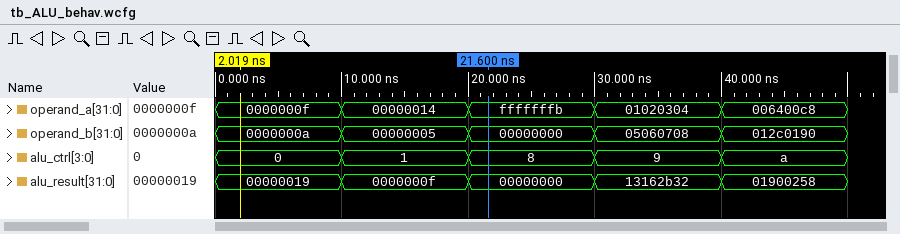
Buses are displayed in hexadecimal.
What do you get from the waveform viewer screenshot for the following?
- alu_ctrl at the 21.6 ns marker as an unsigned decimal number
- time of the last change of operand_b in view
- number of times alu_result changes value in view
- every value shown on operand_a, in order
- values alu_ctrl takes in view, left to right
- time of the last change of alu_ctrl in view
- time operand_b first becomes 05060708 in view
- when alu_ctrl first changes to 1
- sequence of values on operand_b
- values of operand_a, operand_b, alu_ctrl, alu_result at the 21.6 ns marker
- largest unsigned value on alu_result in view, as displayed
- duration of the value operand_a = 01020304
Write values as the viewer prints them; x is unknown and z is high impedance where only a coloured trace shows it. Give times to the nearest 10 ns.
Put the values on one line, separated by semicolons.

8; 40 ns; 4; 0000000f, 00000014, fffffffb, 01020304, 006400c8; 0, 1, 8, 9, a; 40 ns; 30 ns; 10 ns; 0000000a, 00000005, 00000000, 05060708, 012c0190; operand_a=fffffffb, operand_b=00000000, alu_ctrl=8, alu_result=00000000; 13162b32; 10 ns
